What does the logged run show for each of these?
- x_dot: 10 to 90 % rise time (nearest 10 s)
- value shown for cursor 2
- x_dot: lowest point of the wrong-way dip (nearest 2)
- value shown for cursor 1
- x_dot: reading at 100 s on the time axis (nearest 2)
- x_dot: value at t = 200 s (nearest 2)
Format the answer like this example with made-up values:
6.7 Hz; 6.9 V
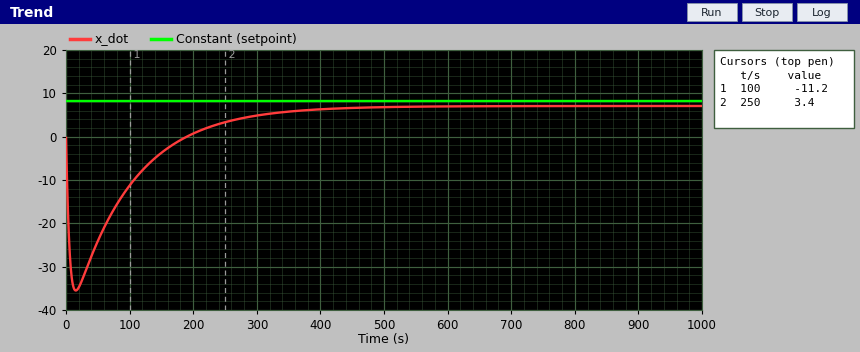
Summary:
210 s; 3.4; -36; -11.2; -12; 0
